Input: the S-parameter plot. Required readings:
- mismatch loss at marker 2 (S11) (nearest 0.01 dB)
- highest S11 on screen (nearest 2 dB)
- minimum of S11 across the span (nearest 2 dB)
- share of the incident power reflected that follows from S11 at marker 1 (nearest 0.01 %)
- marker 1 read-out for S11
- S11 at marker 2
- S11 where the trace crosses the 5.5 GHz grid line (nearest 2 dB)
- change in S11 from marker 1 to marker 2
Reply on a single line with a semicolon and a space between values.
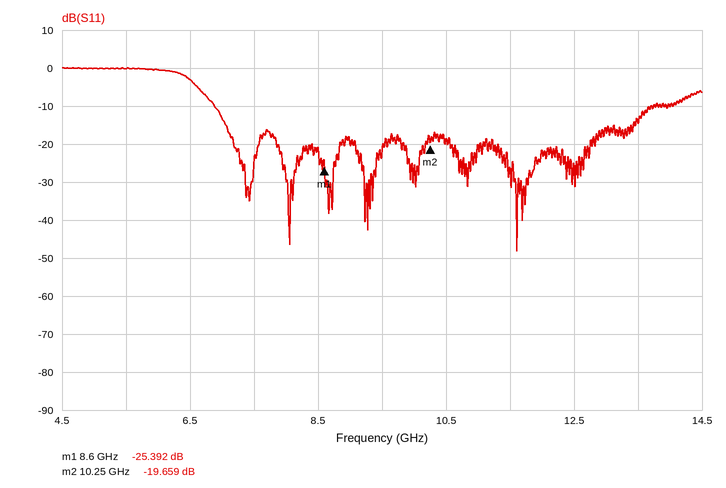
0.05 dB; 0 dB; -48 dB; 0.29 %; -25.392 dB; -19.659 dB; 0 dB; 5.733 dB
